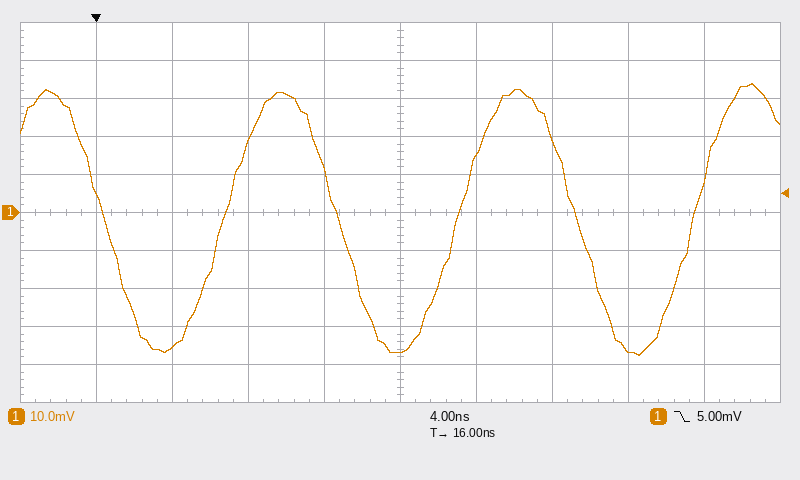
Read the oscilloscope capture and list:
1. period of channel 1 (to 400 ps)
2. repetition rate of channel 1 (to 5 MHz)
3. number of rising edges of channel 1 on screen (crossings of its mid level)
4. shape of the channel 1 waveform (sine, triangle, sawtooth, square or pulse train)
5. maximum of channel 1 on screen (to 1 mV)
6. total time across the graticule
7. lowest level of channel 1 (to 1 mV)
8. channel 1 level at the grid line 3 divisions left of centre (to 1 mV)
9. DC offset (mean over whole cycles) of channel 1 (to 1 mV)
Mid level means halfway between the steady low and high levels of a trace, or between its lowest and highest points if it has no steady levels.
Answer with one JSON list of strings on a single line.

["12.4 ns", "80 MHz", "3", "sine", "34 mV", "40 ns", "-38 mV", "-35 mV", "-2 mV"]
